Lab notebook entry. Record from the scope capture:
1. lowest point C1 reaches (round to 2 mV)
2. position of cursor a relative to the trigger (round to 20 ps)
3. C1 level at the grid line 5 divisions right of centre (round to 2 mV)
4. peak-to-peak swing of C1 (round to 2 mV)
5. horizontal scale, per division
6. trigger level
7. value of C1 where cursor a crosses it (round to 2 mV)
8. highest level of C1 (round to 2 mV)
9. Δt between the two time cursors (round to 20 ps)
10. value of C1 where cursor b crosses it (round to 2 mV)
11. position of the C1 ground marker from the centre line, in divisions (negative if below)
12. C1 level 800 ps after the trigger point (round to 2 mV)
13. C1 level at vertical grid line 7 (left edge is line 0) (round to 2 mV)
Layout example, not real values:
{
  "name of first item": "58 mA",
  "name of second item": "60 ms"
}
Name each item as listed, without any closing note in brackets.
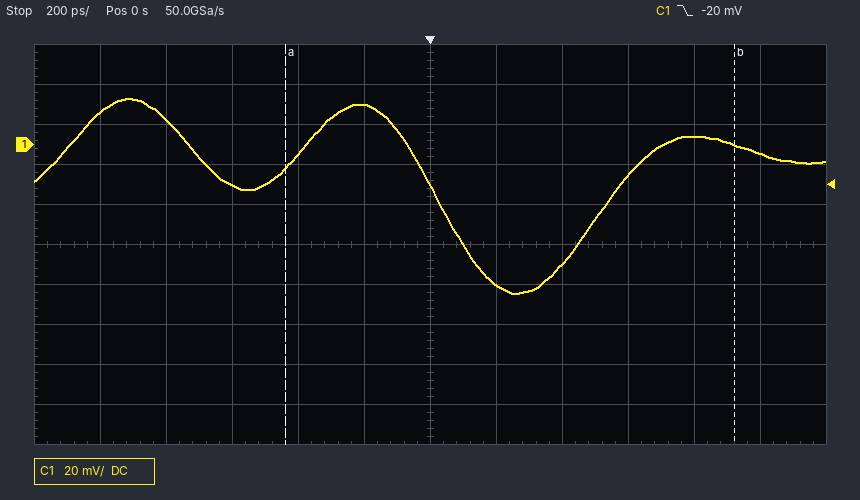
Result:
{
  "lowest point C1 reaches": "-74 mV",
  "position of cursor a relative to the trigger": "-440 ps",
  "C1 level at the grid line 5 divisions right of centre": "-4 mV",
  "peak-to-peak swing of C1": "98 mV",
  "horizontal scale, per division": "200 ps",
  "trigger level": "-20 mV",
  "value of C1 where cursor a crosses it": "-12 mV",
  "highest level of C1": "24 mV",
  "Δt between the two time cursors": "1.36 ns",
  "value of C1 where cursor b crosses it": "0 mV",
  "position of the C1 ground marker from the centre line, in divisions": "+2.5 div",
  "C1 level 800 ps after the trigger point": "4 mV",
  "C1 level at vertical grid line 7 (left edge is line 0)": "-70 mV"
}
